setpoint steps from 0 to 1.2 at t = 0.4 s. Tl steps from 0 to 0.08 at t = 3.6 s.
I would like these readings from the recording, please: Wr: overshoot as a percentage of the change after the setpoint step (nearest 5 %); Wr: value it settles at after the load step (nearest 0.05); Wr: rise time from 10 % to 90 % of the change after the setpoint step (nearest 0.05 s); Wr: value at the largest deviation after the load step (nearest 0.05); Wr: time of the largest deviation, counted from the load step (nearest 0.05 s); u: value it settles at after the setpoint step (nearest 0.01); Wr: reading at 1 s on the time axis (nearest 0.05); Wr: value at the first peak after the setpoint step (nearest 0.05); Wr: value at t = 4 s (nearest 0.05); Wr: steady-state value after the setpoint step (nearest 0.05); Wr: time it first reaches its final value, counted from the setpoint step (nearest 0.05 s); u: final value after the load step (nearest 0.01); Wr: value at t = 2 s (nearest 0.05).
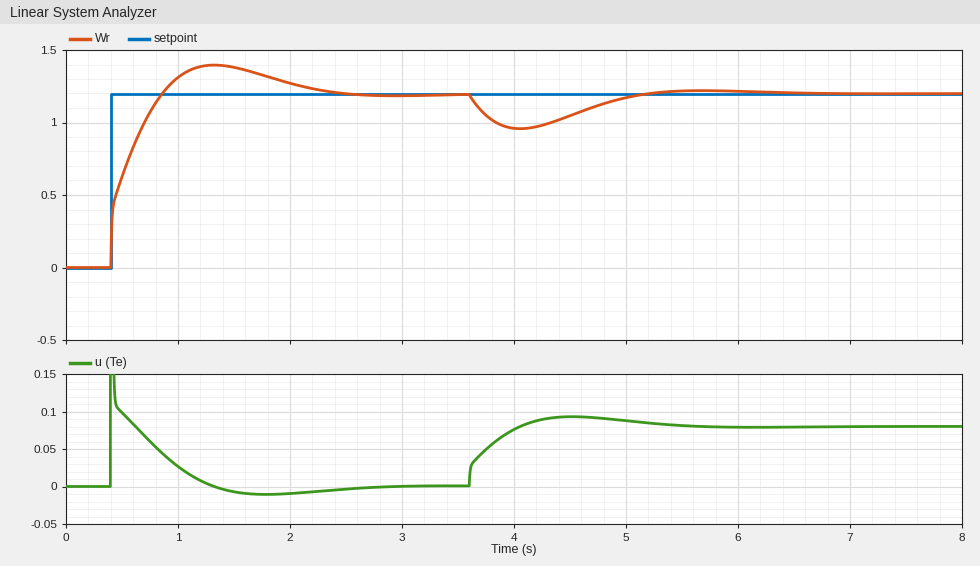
15 %
1.20
0.35 s
0.95
0.45 s
0.00
1.30
1.40
0.95
1.20
0.45 s
0.08
1.25
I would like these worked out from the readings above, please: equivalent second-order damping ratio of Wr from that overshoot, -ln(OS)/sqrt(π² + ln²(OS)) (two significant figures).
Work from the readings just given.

0.52
